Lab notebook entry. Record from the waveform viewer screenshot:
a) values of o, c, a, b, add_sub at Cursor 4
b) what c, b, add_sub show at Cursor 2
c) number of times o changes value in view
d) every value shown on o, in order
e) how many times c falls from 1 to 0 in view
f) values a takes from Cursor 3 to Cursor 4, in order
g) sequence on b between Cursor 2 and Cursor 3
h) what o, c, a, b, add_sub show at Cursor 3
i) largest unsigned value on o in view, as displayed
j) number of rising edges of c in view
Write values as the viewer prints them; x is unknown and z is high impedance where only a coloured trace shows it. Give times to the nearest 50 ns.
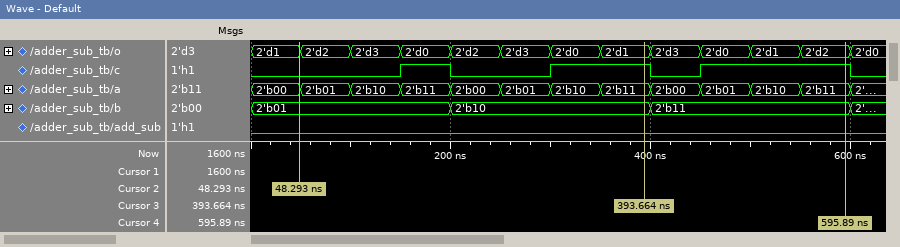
o=2'd2, c=1, a=2'b11, b=2'b11, add_sub=0
c=0, b=2'b01, add_sub=0
12
2'd1, 2'd2, 2'd3, 2'd0, 2'd2, 2'd3, 2'd0, 2'd1, 2'd3, 2'd0, 2'd1, 2'd2, 2'd0
3
2'b11, 2'b00, 2'b01, 2'b10, 2'b11
2'b01, 2'b10
o=2'd1, c=1, a=2'b11, b=2'b10, add_sub=0
2'd3
3
